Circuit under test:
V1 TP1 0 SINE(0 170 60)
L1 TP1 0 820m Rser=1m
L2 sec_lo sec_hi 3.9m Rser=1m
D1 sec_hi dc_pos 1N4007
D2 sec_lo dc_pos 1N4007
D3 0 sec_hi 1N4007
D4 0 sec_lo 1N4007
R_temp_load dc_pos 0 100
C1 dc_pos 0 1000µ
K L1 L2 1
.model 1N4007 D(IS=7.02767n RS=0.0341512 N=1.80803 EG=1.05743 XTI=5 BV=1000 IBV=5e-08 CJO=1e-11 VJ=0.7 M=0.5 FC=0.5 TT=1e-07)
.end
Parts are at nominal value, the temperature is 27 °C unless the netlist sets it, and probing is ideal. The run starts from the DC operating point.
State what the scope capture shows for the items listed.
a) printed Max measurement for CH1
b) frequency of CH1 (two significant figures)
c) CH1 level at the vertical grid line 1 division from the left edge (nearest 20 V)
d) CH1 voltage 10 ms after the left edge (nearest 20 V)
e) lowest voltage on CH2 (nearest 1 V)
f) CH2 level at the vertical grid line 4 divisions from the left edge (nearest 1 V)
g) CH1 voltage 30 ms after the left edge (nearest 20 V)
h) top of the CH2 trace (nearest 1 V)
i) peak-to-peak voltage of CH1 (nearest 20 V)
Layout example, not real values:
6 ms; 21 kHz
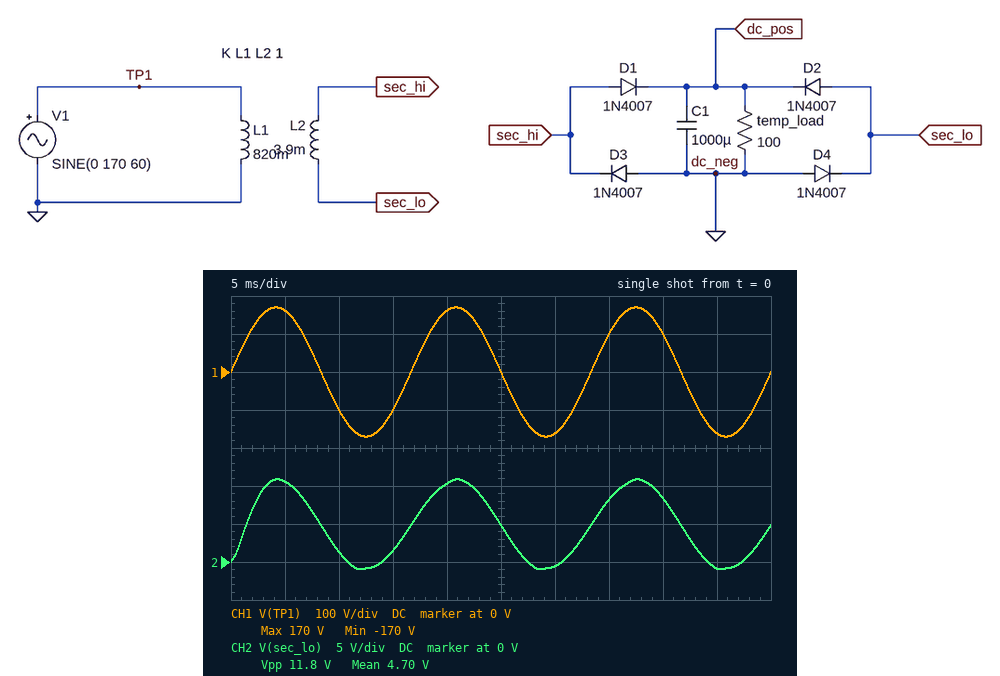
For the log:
170 V; 60 Hz; 160 V; -100 V; -1 V; 10 V; -160 V; 11 V; 340 V
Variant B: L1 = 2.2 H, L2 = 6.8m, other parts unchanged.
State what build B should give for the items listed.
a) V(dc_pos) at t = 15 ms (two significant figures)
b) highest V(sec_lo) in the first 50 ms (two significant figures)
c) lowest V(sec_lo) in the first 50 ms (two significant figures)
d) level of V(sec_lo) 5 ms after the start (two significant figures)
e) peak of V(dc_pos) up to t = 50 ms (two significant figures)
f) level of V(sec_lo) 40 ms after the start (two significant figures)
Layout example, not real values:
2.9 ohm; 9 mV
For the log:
7.7 V; 8.6 V; -890 mV; 8.4 V; 7.8 V; 6.6 V
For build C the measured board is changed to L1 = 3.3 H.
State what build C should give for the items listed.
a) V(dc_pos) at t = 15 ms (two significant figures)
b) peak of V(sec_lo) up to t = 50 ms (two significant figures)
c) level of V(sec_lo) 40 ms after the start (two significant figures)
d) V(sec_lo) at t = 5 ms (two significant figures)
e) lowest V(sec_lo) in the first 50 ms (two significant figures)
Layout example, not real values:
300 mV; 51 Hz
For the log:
4.2 V; 5.0 V; 3.8 V; 4.9 V; -840 mV
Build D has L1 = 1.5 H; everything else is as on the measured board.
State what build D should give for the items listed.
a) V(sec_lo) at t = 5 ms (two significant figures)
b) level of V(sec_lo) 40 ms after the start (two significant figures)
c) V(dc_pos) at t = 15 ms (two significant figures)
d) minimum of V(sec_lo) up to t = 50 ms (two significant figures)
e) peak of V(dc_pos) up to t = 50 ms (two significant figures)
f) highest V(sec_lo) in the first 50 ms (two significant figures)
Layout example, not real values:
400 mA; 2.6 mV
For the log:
7.6 V; 6.0 V; 6.9 V; -880 mV; 7.0 V; 7.8 V
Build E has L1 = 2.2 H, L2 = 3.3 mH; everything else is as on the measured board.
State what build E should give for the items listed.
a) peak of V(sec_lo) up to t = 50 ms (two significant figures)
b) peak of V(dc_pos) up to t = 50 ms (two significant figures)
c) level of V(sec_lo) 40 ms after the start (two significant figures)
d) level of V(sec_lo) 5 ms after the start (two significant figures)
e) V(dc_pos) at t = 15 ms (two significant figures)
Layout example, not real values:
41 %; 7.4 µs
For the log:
5.8 V; 5.0 V; 4.4 V; 5.6 V; 4.9 V
